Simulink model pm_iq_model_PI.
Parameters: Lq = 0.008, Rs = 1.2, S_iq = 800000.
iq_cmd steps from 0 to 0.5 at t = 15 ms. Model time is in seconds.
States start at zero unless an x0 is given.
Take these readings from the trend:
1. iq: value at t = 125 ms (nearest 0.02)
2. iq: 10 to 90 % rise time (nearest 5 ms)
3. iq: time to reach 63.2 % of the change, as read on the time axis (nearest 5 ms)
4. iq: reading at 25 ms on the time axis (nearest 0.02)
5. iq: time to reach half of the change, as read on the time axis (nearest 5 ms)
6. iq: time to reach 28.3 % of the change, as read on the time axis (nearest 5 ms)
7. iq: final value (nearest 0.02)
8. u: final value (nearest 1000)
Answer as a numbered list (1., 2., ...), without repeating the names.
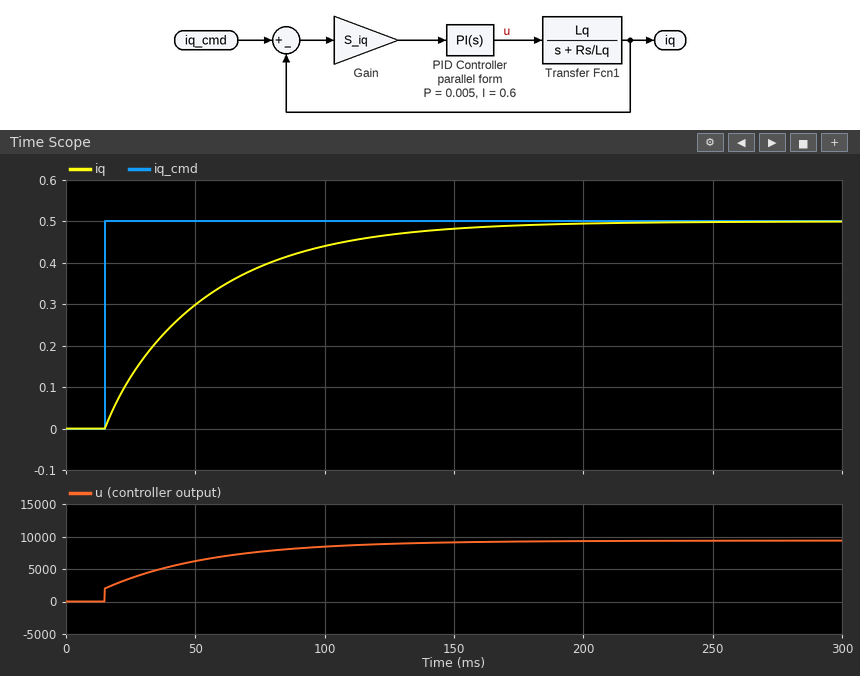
1. 0.46
2. 90 ms
3. 55 ms
4. 0.12
5. 40 ms
6. 25 ms
7. 0.50
8. 9000
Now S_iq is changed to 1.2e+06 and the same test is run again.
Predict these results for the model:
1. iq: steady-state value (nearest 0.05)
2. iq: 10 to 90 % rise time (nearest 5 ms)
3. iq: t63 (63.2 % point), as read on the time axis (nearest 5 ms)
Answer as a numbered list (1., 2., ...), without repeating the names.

1. 0.50
2. 60 ms
3. 40 ms
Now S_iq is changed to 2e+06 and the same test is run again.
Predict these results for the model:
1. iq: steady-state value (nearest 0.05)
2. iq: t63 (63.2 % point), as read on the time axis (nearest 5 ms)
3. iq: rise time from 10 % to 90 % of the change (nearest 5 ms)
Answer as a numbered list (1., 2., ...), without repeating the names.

1. 0.50
2. 30 ms
3. 35 ms
